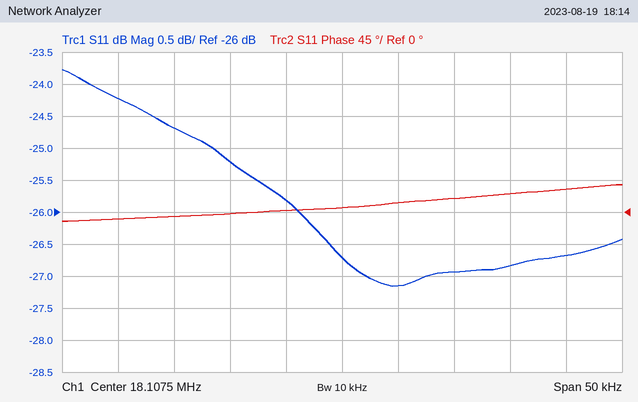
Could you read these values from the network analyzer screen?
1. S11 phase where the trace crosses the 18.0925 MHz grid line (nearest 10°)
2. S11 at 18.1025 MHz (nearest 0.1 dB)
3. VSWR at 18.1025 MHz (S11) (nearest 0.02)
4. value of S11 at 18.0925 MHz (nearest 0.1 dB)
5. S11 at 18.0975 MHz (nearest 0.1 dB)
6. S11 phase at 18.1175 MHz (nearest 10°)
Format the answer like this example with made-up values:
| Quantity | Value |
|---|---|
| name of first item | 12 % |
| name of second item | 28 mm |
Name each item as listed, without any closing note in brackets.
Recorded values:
| Quantity | Value |
|---|---|
| S11 phase where the trace crosses the 18.0925 MHz grid line | -10° |
| S11 at 18.1025 MHz | -25.8 dB |
| VSWR at 18.1025 MHz (S11) | 1.10 |
| value of S11 at 18.0925 MHz | -24.7 dB |
| S11 at 18.0975 MHz | -25.2 dB |
| S11 phase at 18.1175 MHz | 20° |
